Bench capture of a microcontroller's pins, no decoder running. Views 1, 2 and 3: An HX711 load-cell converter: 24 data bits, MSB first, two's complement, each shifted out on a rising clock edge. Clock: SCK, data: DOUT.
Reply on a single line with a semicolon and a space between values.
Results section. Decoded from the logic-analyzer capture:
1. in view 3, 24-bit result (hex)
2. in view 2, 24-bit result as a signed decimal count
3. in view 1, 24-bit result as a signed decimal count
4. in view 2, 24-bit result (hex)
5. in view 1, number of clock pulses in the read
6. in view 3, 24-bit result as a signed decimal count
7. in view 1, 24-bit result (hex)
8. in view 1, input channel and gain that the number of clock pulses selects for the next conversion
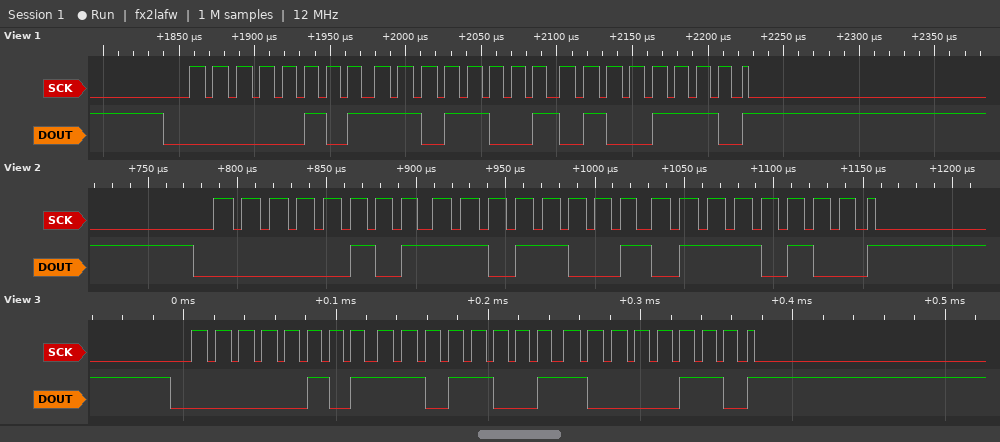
0x05D986; 383348; 383310; 0x05D974; 25; 383366; 0x05D94E; channel A, gain 128
